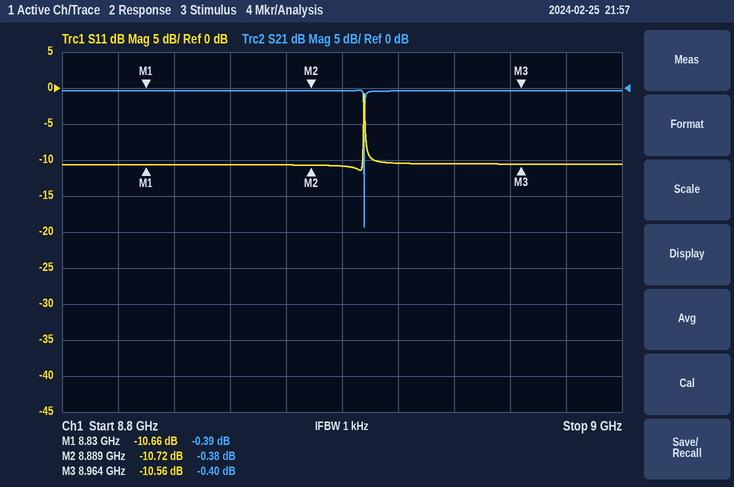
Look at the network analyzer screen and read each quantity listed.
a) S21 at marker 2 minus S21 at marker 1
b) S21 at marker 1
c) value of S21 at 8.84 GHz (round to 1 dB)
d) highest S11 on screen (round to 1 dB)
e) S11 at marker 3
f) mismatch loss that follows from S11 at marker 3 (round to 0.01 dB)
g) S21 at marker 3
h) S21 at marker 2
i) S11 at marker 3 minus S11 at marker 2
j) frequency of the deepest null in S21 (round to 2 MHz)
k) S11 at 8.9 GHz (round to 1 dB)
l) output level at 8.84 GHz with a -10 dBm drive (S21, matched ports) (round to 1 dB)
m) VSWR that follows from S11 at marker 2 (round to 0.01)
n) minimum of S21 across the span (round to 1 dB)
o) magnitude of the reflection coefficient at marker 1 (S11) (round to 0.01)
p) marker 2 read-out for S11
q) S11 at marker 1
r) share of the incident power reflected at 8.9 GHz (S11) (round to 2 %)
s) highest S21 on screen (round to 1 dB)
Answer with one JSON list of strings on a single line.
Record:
["0.01 dB", "-0.39 dB", "0 dB", "-1 dB", "-10.56 dB", "0.40 dB", "-0.40 dB", "-0.38 dB", "0.16 dB", "8.908 GHz", "-11 dB", "-10 dBm", "1.82", "-19 dB", "0.29", "-10.72 dB", "-10.66 dB", "8 %", "0 dB"]
